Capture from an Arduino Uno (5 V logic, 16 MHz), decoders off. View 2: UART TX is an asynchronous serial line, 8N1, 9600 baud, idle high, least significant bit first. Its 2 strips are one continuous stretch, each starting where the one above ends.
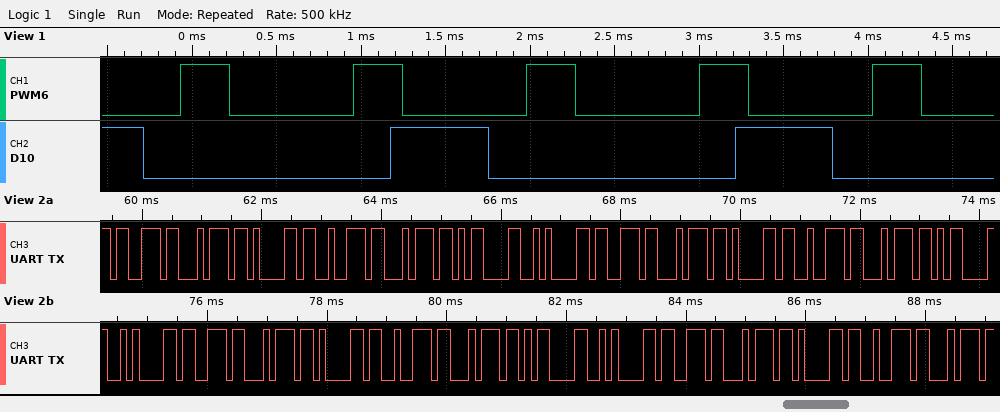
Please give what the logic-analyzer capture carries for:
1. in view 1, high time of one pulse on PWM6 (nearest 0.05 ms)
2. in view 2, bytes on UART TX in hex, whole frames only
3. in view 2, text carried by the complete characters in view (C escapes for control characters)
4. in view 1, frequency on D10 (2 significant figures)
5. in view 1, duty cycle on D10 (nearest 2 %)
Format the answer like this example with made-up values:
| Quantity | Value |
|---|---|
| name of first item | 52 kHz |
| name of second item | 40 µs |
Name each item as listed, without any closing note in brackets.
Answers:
| Quantity | Value |
|---|---|
| in view 1, high time of one pulse on PWM6 | 0.30 ms |
| in view 2, bytes on UART TX in hex, whole frames only | 73 74 61 72 74 0D 0A 73 74 61 72 74 0D 0A 73 74 61 72 74 0D 0A 73 74 61 72 74 |
| in view 2, text carried by the complete characters in view | "start\r\nstart\r\nstart\r\nstart" |
| in view 1, frequency on D10 | 490 Hz |
| in view 1, duty cycle on D10 | 28 % |
